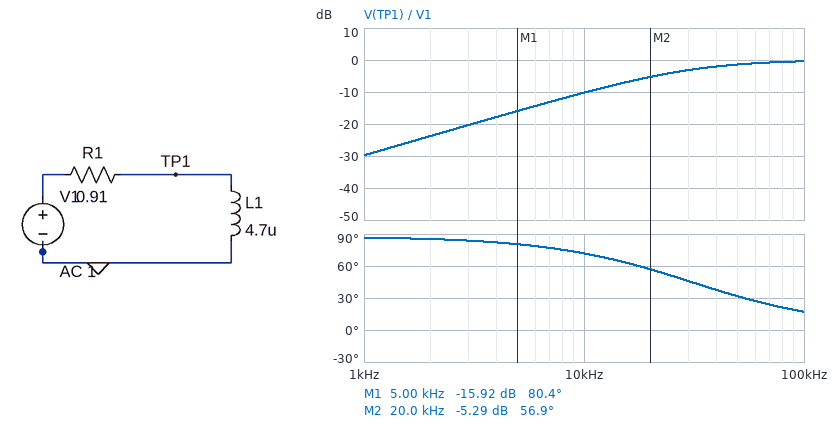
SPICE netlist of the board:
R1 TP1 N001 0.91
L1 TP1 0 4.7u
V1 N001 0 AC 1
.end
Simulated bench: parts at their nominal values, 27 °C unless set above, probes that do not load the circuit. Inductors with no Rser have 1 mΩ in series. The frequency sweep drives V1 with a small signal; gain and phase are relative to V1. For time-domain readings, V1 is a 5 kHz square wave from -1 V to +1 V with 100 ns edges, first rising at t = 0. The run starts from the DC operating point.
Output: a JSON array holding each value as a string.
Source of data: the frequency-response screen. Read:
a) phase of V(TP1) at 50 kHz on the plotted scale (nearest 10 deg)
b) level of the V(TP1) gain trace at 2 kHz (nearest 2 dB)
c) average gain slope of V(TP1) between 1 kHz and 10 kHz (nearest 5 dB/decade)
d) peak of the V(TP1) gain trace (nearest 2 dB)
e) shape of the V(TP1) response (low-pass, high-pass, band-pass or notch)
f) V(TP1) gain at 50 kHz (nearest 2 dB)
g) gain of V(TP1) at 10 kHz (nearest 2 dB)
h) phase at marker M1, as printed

["30 deg", "-24 dB", "20 dB/decade", "0 dB", "high-pass", "-2 dB", "-10 dB", "80.4 deg"]
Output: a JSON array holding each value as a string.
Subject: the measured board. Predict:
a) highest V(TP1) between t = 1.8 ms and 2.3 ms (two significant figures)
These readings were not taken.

["2.0 V"]
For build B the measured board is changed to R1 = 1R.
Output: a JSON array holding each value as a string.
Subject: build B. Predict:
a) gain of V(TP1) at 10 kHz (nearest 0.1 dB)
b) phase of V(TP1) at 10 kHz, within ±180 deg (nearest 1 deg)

["-11.0 dB", "73 deg"]
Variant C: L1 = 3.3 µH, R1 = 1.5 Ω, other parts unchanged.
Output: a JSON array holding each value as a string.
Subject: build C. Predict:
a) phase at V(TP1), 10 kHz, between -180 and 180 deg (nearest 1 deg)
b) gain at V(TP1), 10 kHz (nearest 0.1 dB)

["82 deg", "-17.3 dB"]
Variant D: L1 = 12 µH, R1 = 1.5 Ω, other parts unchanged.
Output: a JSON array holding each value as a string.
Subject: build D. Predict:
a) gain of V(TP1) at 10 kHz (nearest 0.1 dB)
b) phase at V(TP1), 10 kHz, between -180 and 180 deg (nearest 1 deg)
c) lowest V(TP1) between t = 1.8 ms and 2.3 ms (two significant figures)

["-7.0 dB", "63 deg", "-2.0 V"]
